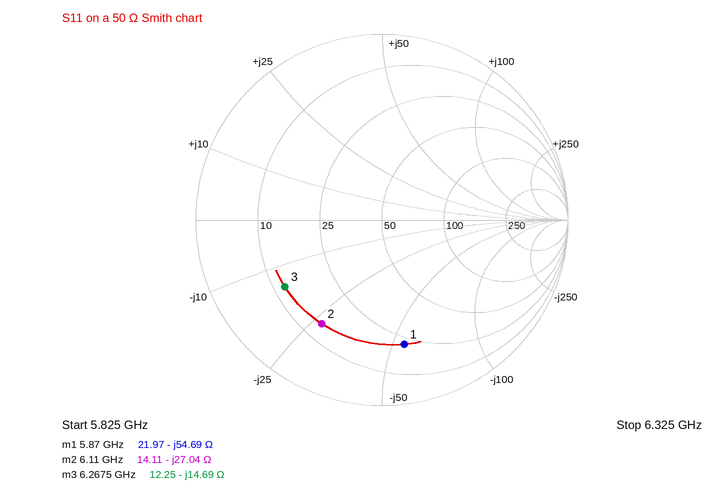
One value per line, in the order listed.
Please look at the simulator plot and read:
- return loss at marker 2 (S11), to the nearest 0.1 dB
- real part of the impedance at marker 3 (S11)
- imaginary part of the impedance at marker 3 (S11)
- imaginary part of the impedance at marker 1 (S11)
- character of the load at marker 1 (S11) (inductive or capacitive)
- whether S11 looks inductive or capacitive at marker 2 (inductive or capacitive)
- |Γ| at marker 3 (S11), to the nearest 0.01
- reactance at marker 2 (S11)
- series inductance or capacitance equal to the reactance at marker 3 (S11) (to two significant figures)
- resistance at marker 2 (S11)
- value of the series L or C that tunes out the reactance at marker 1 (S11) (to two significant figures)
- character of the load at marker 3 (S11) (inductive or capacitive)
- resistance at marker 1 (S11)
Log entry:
3.8 dB
12.25 Ω
-14.69 Ω
-54.69 Ω
capacitive
capacitive
0.63
-27.04 Ω
1.7 pF
14.11 Ω
1.5 nH
capacitive
21.97 Ω
